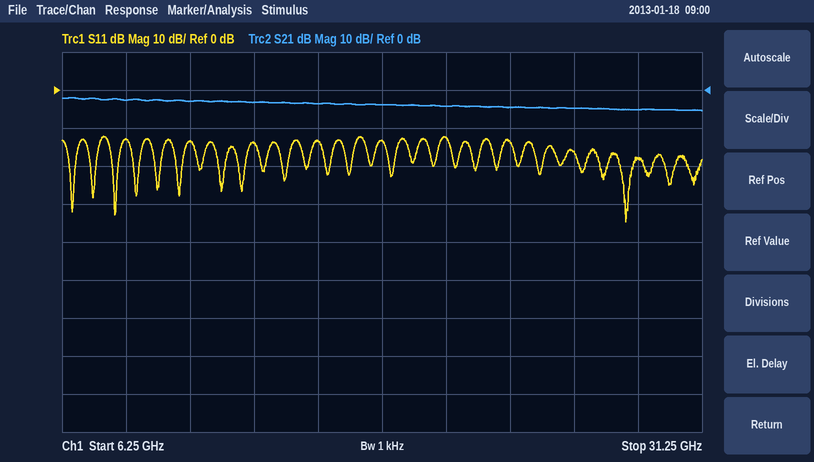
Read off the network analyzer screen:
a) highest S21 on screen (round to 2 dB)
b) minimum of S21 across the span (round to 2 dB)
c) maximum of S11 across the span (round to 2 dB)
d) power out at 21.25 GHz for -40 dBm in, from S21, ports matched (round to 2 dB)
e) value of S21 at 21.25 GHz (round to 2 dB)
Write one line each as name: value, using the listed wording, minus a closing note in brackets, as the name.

highest S21 on screen: -2 dB
minimum of S21 across the span: -6 dB
maximum of S11 across the span: -12 dB
power out at 21.25 GHz for -40 dBm in, from S21, ports matched: -44 dBm
value of S21 at 21.25 GHz: -4 dB
